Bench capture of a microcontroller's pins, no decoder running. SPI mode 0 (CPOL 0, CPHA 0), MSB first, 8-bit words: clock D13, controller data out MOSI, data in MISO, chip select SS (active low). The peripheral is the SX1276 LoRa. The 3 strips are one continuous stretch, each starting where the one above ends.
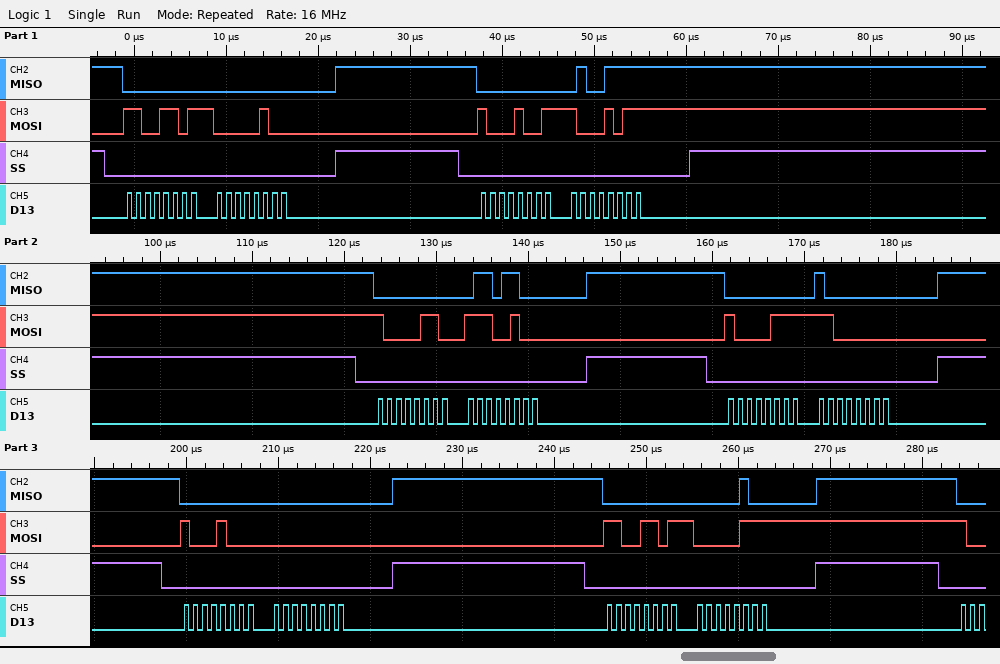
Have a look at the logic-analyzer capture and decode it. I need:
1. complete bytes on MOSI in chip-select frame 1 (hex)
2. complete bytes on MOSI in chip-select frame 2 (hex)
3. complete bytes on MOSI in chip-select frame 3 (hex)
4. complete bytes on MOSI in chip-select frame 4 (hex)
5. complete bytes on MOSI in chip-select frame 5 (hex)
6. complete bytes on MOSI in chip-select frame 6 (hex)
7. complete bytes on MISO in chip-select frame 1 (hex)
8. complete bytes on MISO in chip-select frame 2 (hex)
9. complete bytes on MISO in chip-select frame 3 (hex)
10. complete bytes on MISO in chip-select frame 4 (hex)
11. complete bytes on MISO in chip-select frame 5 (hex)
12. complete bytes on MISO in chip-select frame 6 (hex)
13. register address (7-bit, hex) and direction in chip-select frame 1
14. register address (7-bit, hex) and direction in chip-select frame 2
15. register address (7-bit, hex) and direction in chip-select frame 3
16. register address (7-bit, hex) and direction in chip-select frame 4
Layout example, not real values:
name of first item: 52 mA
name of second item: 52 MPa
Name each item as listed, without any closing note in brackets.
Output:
complete bytes on MOSI in chip-select frame 1: CD 04
complete bytes on MOSI in chip-select frame 2: 89 8B
complete bytes on MOSI in chip-select frame 3: 86 E4
complete bytes on MOSI in chip-select frame 4: 87 C0
complete bytes on MOSI in chip-select frame 5: 88 00
complete bytes on MOSI in chip-select frame 6: CD 07
complete bytes on MISO in chip-select frame 1: 00 00
complete bytes on MISO in chip-select frame 2: 00 4F
complete bytes on MISO in chip-select frame 3: 00 6C
complete bytes on MISO in chip-select frame 4: 00 80
complete bytes on MISO in chip-select frame 5: 00 00
complete bytes on MISO in chip-select frame 6: 00 04
register address (7-bit, hex) and direction in chip-select frame 1: 0x4D write
register address (7-bit, hex) and direction in chip-select frame 2: 0x09 write
register address (7-bit, hex) and direction in chip-select frame 3: 0x06 write
register address (7-bit, hex) and direction in chip-select frame 4: 0x07 write
